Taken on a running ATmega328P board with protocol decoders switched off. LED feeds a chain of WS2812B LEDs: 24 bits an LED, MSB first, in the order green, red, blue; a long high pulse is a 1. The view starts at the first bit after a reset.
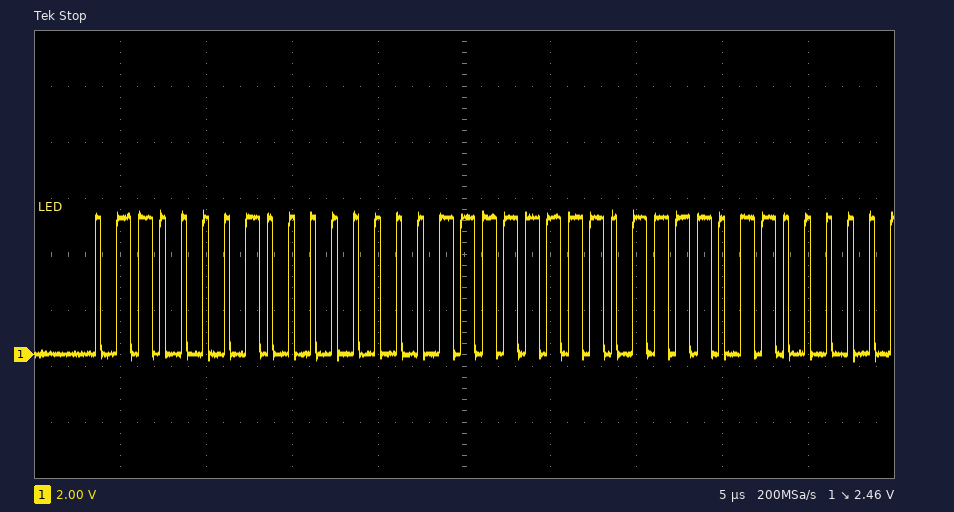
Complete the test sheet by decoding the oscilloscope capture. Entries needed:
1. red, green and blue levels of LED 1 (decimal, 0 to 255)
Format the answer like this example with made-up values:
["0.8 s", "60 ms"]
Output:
["0, 97, 255"]
